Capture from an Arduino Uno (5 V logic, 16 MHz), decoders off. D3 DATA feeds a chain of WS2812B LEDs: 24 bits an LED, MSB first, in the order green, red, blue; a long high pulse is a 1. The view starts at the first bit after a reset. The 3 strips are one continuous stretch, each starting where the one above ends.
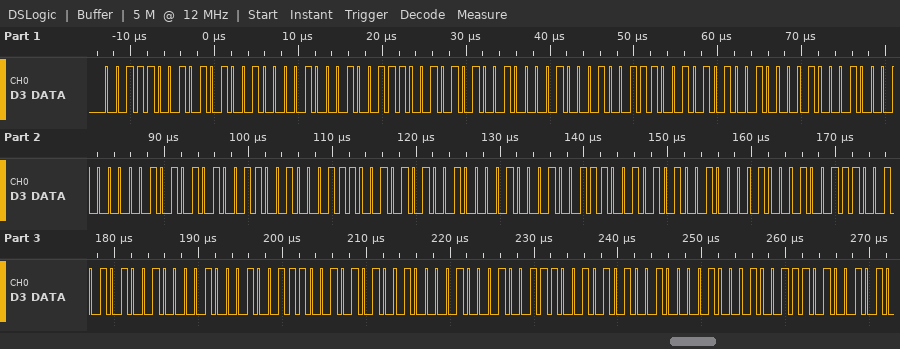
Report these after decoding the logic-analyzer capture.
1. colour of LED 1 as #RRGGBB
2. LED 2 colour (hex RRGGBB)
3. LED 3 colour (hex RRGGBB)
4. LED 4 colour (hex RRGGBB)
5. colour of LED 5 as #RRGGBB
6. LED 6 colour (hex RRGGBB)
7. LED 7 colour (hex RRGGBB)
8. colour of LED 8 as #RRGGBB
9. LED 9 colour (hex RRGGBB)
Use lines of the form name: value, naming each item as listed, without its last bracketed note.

colour of LED 1 as #RRGGBB: #523911
LED 2 colour: #523911
LED 3 colour: #523911
LED 4 colour: #550032
colour of LED 5 as #RRGGBB: #523911
LED 6 colour: #523911
LED 7 colour: #523911
colour of LED 8 as #RRGGBB: #523911
LED 9 colour: #523911
